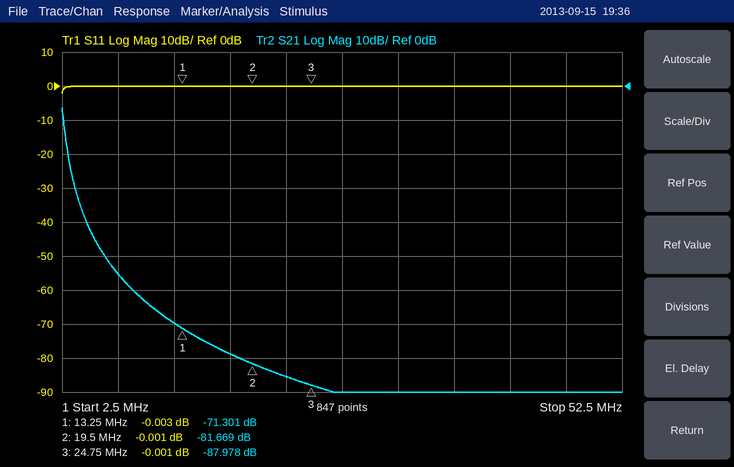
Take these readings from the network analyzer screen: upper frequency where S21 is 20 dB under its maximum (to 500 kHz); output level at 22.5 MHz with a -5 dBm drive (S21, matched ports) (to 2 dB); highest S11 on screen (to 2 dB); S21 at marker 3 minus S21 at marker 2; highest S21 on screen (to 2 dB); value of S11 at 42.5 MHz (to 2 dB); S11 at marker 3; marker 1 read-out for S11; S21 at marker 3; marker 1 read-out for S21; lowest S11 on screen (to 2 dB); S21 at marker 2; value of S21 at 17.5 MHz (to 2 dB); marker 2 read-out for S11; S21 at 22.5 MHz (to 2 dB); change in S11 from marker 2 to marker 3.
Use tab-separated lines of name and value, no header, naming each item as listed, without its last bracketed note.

upper frequency where S21 is 20 dB under its maximum	3.5 MHz
output level at 22.5 MHz with a -5 dBm drive (S21, matched ports)	-90 dBm
highest S11 on screen	0 dB
S21 at marker 3 minus S21 at marker 2	-6.309 dB
highest S21 on screen	-6 dB
value of S11 at 42.5 MHz	0 dB
S11 at marker 3	-0.001 dB
marker 1 read-out for S11	-0.003 dB
S21 at marker 3	-87.978 dB
marker 1 read-out for S21	-71.301 dB
lowest S11 on screen	-2 dB
S21 at marker 2	-81.669 dB
value of S21 at 17.5 MHz	-78 dB
marker 2 read-out for S11	-0.001 dB
S21 at 22.5 MHz	-86 dB
change in S11 from marker 2 to marker 3	0.000 dB
